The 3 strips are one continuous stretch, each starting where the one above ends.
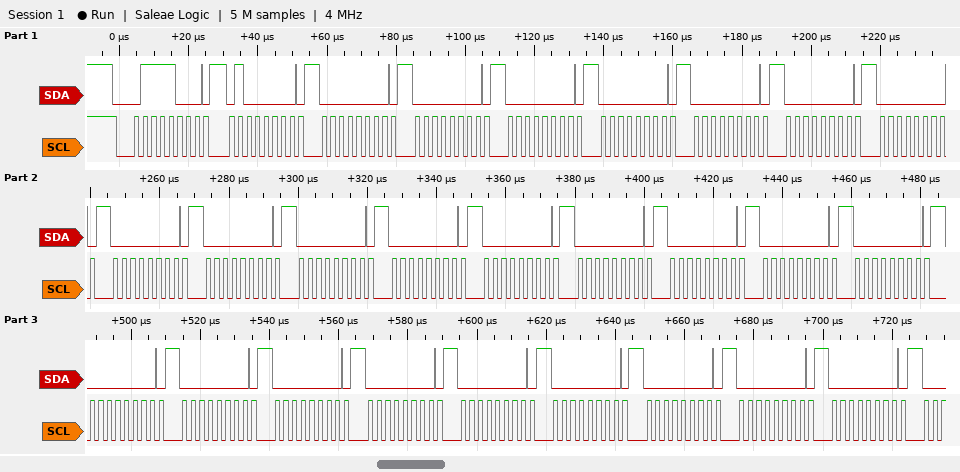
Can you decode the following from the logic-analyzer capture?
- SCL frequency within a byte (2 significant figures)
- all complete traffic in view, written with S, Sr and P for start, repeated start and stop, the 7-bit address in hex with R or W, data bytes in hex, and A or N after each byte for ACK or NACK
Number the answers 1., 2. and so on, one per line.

1. 400 kHz
2. S 3CW A 40 A 00 A 00 A 00 A 00 A 00 A 00 A 00 A 00 A 00 A 00 A 00 A 00 A 00 A 00 A 00 A 00 A 00 A 00 A 00 A 00 A 00 A 00 A 00 A 00 A 00 A
